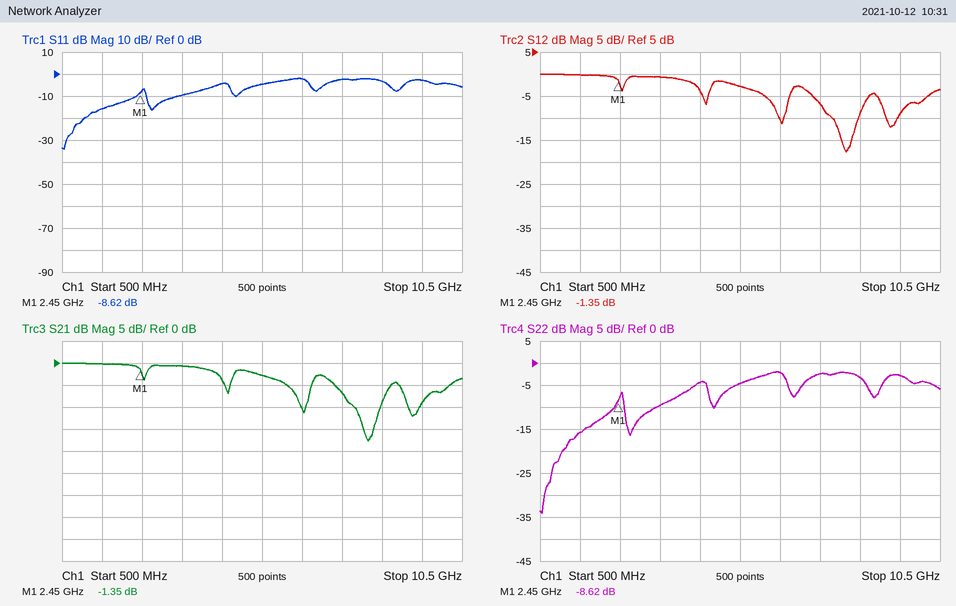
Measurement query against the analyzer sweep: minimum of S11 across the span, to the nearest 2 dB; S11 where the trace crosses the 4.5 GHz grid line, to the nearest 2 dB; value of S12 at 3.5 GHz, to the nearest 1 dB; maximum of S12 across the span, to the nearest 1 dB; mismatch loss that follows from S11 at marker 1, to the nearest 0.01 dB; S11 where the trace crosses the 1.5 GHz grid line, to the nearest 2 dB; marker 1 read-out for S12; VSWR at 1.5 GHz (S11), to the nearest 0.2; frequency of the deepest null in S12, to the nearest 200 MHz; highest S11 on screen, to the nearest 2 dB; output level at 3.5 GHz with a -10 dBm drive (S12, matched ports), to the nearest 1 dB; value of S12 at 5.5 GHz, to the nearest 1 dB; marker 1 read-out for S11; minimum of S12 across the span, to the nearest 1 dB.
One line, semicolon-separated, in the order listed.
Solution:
-34 dB; -4 dB; -1 dB; 0 dB; 0.64 dB; -16 dB; -1.35 dB; 1.4; 8.2 GHz; -2 dB; -11 dBm; -3 dB; -8.62 dB; -18 dB
